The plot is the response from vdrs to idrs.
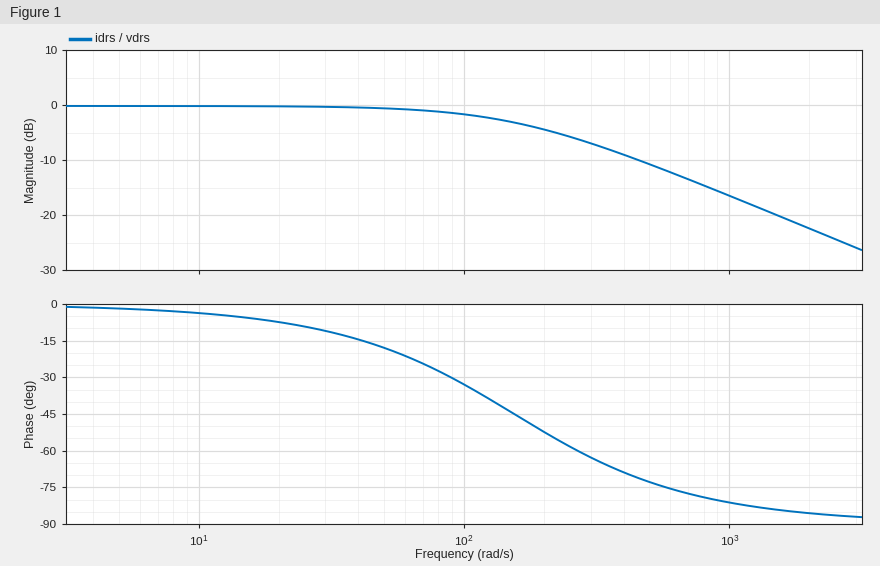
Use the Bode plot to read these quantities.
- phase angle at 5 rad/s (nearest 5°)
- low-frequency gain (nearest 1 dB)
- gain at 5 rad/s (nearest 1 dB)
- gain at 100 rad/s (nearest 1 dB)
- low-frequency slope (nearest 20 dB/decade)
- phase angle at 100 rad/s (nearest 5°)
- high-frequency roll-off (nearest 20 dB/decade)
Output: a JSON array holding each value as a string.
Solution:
["0°", "0 dB", "0 dB", "-2 dB", "0 dB/decade", "-35°", "-20 dB/decade"]
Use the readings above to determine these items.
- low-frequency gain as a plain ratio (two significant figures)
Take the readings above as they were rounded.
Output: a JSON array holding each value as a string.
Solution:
["1.0"]
